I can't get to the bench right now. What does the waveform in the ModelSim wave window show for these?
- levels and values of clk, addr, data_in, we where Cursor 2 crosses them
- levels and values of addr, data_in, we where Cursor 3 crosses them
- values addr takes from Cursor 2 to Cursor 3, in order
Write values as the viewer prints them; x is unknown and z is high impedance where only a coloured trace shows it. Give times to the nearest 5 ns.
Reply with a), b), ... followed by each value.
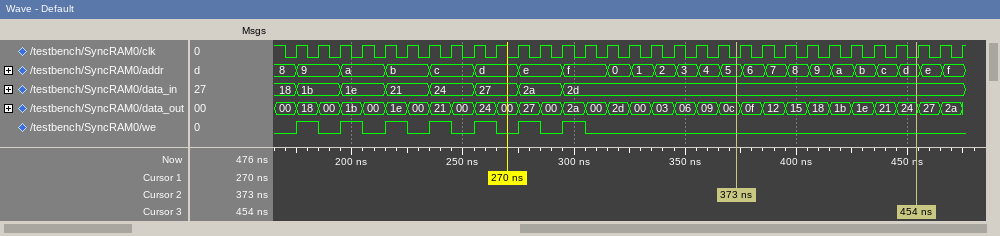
a) clk=0, addr=5, data_in=2d, we=0
b) addr=d, data_in=2d, we=0
c) 5, 6, 7, 8, 9, a, b, c, d
